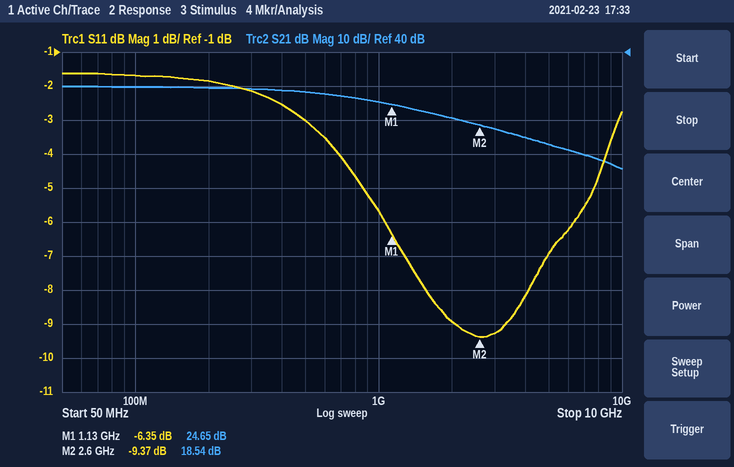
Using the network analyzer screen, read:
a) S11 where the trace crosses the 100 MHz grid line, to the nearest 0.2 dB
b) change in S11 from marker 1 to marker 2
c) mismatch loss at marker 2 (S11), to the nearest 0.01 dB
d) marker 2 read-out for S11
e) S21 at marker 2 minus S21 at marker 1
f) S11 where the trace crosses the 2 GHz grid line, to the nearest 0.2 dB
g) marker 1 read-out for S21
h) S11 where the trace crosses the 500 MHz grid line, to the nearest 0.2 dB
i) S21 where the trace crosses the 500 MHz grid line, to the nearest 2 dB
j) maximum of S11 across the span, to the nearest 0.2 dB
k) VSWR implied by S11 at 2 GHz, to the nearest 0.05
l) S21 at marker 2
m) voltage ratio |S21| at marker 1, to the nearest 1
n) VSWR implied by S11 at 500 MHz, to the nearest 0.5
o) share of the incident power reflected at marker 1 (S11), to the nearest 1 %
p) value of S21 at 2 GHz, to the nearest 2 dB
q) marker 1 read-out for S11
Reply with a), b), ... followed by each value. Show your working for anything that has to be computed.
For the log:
a) -1.6 dB
b) -9.37 − (-6.35) = -3.02 dB
c) −10 log10(1 − 10^(-9.37/10)) ≈ 0.53 dB
d) -9.37 dB
e) 18.54 − (24.65) = -6.11 dB
f) -9.0 dB
g) 24.65 dB
h) -3.0 dB
i) 28 dB
j) -1.6 dB
k) |Γ| = 10^(-9/20) = 0.3548; VSWR = (1 + 0.3548)/(1 − 0.3548) ≈ 2.10
l) 18.54 dB
m) 10^(24.65/20) ≈ 17
n) |Γ| = 10^(-3/20) = 0.7079; VSWR = (1 + 0.7079)/(1 − 0.7079) ≈ 5.85, so 6.0 to the nearest 0.5
o) 10^(-6.35/10) ≈ 23 %
p) 20 dB
q) -6.35 dB
